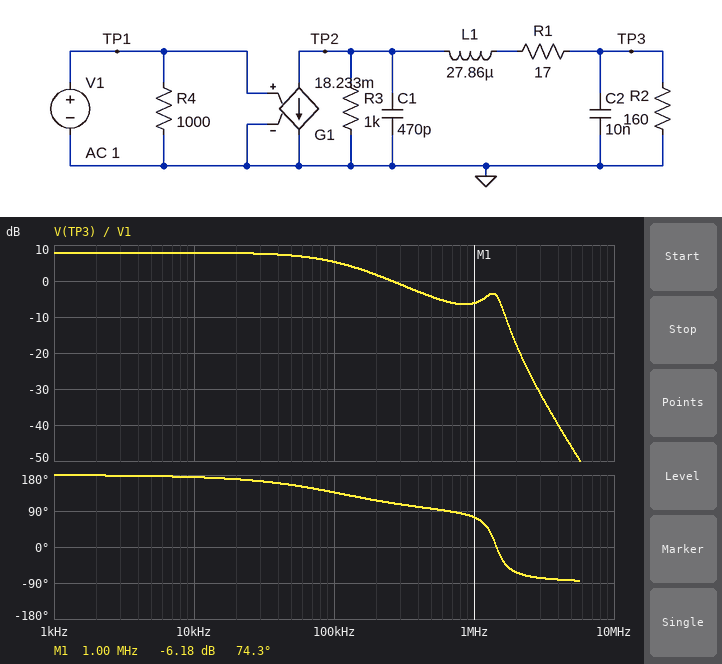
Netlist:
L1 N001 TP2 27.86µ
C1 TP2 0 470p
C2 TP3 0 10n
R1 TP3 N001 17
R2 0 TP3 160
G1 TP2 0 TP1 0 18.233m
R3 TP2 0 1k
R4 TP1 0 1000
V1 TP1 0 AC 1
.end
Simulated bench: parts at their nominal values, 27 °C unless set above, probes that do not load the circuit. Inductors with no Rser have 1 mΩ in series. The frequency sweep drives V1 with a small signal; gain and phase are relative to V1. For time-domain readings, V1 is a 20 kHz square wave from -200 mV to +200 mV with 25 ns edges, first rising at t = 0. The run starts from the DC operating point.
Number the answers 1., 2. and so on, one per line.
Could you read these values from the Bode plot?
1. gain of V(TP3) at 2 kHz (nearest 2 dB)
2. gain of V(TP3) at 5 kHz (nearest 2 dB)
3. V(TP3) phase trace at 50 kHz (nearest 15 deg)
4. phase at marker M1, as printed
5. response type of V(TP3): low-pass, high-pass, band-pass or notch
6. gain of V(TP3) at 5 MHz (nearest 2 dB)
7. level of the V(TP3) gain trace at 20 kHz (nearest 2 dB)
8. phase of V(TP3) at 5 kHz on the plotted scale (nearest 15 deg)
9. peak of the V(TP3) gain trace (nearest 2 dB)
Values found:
1. 8 dB
2. 8 dB
3. 150 deg
4. 74.3 deg
5. low-pass
6. -46 dB
7. 8 dB
8. 180 deg
9. 8 dB
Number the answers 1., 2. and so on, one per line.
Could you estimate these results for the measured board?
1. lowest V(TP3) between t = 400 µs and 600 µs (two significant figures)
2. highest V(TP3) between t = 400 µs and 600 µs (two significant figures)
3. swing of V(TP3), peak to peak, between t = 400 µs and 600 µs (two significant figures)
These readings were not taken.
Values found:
1. -500 mV
2. 500 mV
3. 990 mV
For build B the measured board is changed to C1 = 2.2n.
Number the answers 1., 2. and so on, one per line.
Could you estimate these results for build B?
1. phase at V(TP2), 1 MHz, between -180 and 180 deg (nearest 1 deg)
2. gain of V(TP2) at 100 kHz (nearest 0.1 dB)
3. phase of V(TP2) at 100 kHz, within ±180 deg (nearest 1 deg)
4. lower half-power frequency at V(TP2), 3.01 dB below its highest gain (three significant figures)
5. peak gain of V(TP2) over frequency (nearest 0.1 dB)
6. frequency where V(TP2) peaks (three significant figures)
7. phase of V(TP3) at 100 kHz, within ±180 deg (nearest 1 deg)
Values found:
1. 103 deg
2. 5.0 dB
3. 144 deg
4. 640 kHz
5. 16.1 dB
6. 719 kHz
7. 131 deg
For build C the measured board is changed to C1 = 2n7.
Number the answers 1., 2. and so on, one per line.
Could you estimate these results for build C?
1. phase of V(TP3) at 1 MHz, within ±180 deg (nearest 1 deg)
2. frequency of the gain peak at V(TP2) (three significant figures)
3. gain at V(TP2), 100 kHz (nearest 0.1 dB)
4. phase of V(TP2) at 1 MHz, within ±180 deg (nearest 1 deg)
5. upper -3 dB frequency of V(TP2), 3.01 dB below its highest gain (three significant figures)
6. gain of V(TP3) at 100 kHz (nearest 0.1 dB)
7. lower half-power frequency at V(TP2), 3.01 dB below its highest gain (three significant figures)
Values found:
1. -69 deg
2. 663 kHz
3. 4.8 dB
4. 99 deg
5. 755 kHz
6. 4.6 dB
7. 589 kHz
